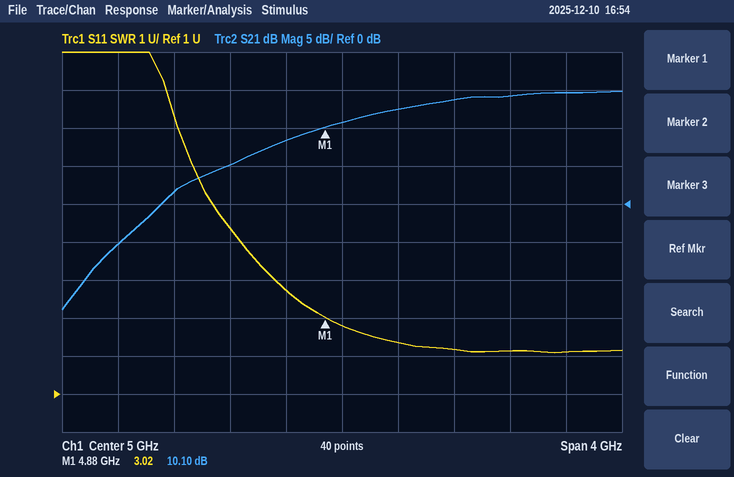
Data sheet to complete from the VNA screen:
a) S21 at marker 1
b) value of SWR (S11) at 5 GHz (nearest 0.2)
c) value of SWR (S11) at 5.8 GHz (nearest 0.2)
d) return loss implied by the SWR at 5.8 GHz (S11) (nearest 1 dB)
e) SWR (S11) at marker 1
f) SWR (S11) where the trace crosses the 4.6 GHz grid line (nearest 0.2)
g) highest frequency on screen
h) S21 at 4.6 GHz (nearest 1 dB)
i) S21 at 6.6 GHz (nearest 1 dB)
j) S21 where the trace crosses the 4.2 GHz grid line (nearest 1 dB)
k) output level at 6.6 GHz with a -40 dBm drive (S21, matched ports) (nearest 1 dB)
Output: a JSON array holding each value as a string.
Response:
["10.10 dB", "2.8", "2.2", "9 dB", "3.02", "3.8", "7 GHz", "8 dB", "15 dB", "5 dB", "-25 dBm"]
